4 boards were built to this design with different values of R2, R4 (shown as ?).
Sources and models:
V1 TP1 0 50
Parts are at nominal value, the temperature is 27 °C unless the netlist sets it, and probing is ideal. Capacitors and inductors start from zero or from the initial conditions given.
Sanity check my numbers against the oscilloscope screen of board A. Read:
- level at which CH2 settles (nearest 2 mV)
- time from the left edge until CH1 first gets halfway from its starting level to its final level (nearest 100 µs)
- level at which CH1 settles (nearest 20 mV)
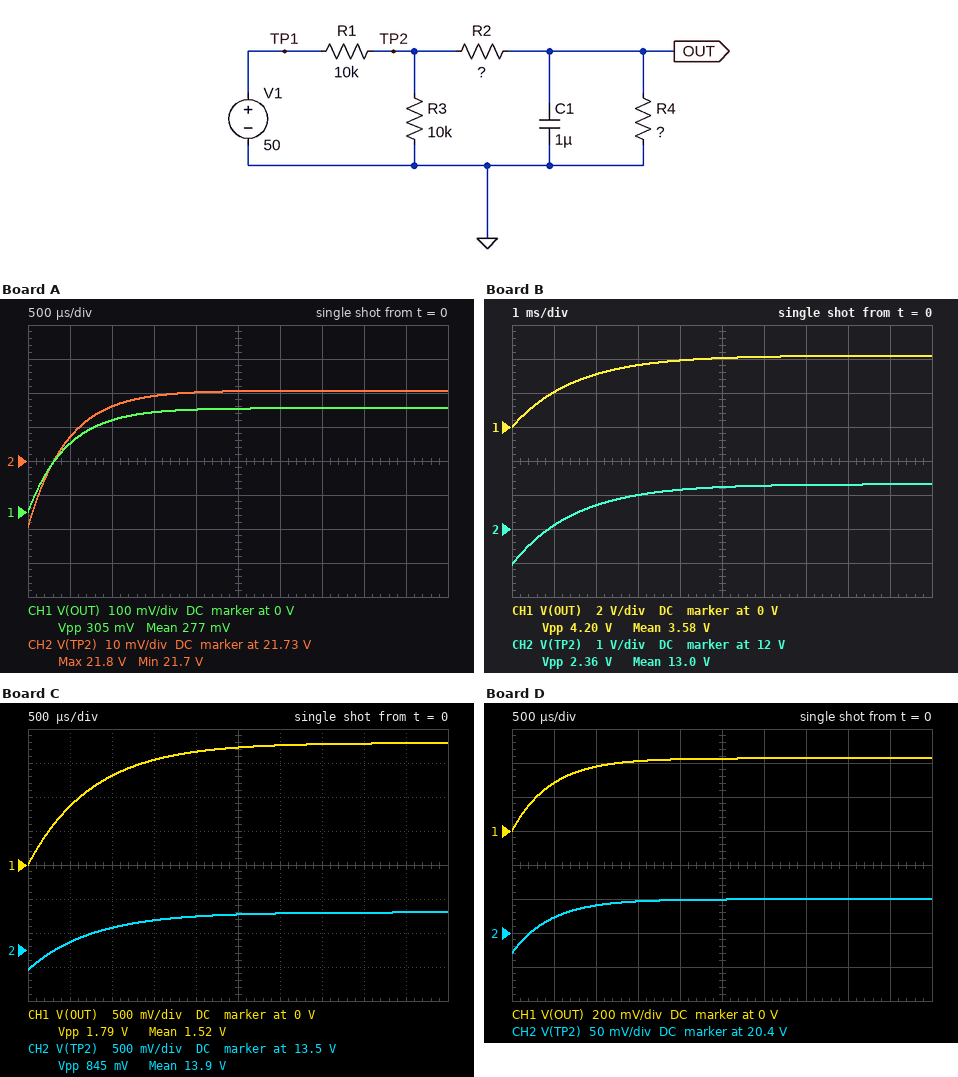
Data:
21.750 V
300 µs
300 mV
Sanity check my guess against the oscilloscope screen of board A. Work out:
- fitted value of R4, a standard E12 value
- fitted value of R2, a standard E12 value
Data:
470 Ω
33 kΩ
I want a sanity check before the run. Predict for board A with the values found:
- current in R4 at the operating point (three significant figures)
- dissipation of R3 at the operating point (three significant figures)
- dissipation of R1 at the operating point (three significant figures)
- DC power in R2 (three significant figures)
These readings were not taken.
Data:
650 µA
47.3 mW
79.8 mW
13.9 mW
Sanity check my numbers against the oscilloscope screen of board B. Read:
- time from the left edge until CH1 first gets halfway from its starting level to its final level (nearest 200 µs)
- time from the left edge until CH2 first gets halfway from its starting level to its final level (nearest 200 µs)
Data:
1.0 ms
1.0 ms
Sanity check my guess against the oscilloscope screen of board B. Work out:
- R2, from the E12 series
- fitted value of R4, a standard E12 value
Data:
3.9 kΩ
1.8 kΩ
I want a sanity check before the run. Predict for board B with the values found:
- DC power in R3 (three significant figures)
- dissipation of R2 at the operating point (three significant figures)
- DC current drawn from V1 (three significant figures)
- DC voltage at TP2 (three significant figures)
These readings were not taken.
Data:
17.7 mW
21.3 mW
3.67 mA
13.3 V
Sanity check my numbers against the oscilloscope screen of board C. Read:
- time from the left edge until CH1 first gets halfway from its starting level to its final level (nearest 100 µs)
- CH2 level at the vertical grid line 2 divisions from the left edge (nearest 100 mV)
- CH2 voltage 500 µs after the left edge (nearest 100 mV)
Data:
500 µs
13.8 V
13.6 V
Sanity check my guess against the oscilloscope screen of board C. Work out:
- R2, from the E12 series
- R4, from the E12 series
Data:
5.6 kΩ
820 Ω
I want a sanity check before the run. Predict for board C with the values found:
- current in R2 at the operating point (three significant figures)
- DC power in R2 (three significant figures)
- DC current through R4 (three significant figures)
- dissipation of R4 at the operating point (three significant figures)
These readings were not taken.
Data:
2.19 mA
26.8 mW
2.19 mA
3.93 mW
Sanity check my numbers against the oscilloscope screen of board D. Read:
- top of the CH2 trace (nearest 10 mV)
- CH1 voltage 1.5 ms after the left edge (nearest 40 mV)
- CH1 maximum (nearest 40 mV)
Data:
20.45 V
400 mV
440 mV
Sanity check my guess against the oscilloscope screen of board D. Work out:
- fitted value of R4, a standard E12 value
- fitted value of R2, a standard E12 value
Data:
470 Ω
22 kΩ
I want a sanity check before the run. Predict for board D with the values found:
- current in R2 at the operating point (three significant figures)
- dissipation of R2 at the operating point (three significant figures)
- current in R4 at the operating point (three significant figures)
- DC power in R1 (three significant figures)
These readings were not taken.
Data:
910 µA
18.2 mW
910 µA
87.3 mW
